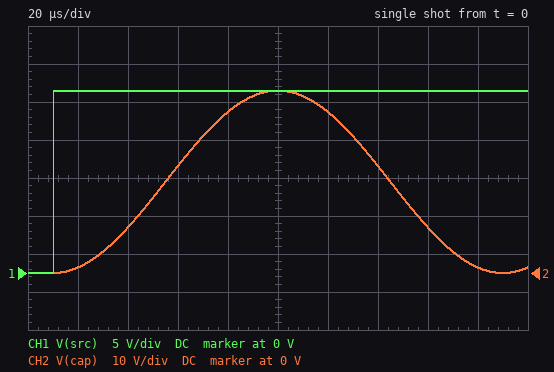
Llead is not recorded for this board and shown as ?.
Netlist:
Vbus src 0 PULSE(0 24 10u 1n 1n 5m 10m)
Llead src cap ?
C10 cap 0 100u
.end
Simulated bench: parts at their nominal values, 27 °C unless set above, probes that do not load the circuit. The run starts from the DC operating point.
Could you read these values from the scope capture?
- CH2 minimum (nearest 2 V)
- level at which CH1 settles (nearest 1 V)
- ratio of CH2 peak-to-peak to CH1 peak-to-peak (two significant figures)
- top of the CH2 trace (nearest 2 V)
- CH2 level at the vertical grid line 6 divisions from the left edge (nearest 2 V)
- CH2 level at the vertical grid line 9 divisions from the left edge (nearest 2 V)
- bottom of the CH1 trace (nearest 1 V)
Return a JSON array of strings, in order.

["0 V", "24 V", "2.0", "48 V", "42 V", "2 V", "0 V"]
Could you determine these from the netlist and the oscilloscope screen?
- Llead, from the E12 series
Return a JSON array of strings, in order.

["8.2 µH"]
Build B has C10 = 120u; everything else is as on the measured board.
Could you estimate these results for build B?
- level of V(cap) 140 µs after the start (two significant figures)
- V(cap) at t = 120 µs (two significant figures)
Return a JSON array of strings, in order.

["37 V", "46 V"]
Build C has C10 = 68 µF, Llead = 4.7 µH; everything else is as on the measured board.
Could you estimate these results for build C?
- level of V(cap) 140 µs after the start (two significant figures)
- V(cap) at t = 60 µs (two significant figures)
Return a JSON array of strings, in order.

["11 V", "47 V"]
